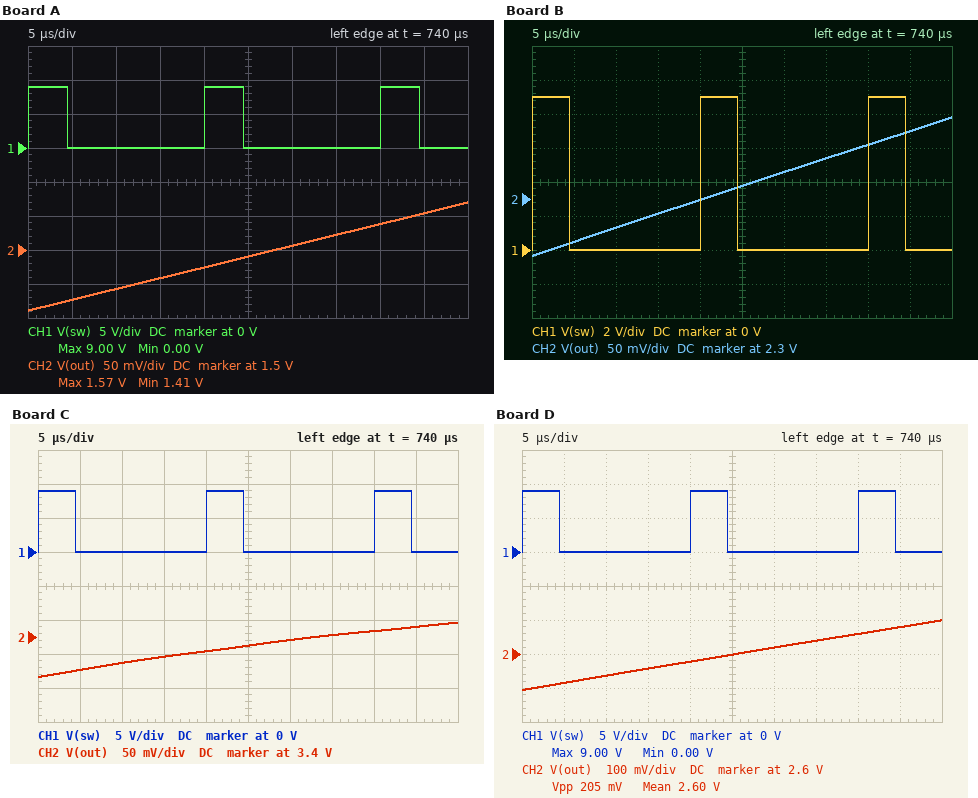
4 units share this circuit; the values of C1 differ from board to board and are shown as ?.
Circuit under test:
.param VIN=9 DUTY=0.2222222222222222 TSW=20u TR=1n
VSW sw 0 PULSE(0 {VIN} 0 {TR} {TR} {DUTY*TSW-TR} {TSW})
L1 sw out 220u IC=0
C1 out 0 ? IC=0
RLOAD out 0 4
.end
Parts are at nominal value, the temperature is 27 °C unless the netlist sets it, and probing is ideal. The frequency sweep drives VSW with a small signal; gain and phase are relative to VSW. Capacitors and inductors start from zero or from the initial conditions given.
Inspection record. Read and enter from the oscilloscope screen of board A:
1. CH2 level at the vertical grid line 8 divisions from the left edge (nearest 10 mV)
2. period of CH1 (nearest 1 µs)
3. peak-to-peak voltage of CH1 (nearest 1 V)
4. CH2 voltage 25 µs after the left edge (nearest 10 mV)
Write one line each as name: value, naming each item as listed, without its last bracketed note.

CH2 level at the vertical grid line 8 divisions from the left edge: 1.54 V
period of CH1: 20 µs
peak-to-peak voltage of CH1: 9 V
CH2 voltage 25 µs after the left edge: 1.49 V
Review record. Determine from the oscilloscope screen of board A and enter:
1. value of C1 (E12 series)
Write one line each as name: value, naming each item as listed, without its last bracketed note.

value of C1: 1.5 mF
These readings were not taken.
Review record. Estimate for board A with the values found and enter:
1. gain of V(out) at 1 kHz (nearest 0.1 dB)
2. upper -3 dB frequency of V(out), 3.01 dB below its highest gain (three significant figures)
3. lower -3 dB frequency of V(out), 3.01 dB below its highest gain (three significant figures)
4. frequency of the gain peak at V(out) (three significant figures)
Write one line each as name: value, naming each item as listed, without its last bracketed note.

gain of V(out) at 1 kHz: -21.6 dB
upper -3 dB frequency of V(out), 3.01 dB below its highest gain: 289 Hz
lower -3 dB frequency of V(out), 3.01 dB below its highest gain: 263 Hz
frequency of the gain peak at V(out): 276 Hz
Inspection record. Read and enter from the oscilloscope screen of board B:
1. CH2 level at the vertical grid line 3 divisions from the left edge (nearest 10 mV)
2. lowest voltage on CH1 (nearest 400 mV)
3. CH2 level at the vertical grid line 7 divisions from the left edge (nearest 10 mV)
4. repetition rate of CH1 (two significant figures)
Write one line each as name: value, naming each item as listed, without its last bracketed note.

CH2 level at the vertical grid line 3 divisions from the left edge: 2.28 V
lowest voltage on CH1: 0 V
CH2 level at the vertical grid line 7 divisions from the left edge: 2.36 V
repetition rate of CH1: 50 kHz
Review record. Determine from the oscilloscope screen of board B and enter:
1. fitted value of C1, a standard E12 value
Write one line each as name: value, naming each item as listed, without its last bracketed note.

fitted value of C1, a standard E12 value: 820 µF
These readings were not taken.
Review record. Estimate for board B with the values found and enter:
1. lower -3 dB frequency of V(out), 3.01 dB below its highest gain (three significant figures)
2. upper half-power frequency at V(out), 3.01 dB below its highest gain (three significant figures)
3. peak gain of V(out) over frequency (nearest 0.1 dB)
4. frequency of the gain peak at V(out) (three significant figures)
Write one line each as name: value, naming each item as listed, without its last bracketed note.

lower -3 dB frequency of V(out), 3.01 dB below its highest gain: 348 Hz
upper half-power frequency at V(out), 3.01 dB below its highest gain: 397 Hz
peak gain of V(out) over frequency: 17.8 dB
frequency of the gain peak at V(out): 373 Hz
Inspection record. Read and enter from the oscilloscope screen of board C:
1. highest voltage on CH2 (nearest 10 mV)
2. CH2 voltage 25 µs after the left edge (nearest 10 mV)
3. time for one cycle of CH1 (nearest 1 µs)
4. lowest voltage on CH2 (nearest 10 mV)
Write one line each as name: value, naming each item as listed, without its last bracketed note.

highest voltage on CH2: 3.42 V
CH2 voltage 25 µs after the left edge: 3.39 V
time for one cycle of CH1: 20 µs
lowest voltage on CH2: 3.34 V
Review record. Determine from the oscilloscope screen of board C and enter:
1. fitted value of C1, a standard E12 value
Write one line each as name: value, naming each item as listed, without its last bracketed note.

fitted value of C1, a standard E12 value: 330 µF
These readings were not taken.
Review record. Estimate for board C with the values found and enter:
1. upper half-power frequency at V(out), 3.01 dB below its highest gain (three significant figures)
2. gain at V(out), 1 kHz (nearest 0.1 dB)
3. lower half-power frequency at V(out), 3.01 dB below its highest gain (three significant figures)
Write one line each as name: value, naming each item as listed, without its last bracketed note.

upper half-power frequency at V(out), 3.01 dB below its highest gain: 642 Hz
gain at V(out), 1 kHz: -5.6 dB
lower half-power frequency at V(out), 3.01 dB below its highest gain: 520 Hz
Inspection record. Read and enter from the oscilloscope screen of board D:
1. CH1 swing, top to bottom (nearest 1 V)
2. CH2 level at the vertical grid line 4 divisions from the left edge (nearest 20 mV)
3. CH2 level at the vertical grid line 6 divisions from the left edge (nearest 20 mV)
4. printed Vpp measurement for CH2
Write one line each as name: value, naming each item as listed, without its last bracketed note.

CH1 swing, top to bottom: 9 V
CH2 level at the vertical grid line 4 divisions from the left edge: 2.58 V
CH2 level at the vertical grid line 6 divisions from the left edge: 2.62 V
printed Vpp measurement for CH2: 205 mV
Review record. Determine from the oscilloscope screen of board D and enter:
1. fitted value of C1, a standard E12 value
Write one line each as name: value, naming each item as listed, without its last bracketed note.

fitted value of C1, a standard E12 value: 680 µF
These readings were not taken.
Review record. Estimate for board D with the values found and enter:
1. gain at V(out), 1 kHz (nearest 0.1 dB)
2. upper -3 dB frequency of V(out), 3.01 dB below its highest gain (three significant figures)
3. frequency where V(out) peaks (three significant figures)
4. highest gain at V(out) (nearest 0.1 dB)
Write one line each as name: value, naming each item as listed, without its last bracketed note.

gain at V(out), 1 kHz: -13.8 dB
upper -3 dB frequency of V(out), 3.01 dB below its highest gain: 438 Hz
frequency where V(out) peaks: 409 Hz
highest gain at V(out): 17.0 dB
